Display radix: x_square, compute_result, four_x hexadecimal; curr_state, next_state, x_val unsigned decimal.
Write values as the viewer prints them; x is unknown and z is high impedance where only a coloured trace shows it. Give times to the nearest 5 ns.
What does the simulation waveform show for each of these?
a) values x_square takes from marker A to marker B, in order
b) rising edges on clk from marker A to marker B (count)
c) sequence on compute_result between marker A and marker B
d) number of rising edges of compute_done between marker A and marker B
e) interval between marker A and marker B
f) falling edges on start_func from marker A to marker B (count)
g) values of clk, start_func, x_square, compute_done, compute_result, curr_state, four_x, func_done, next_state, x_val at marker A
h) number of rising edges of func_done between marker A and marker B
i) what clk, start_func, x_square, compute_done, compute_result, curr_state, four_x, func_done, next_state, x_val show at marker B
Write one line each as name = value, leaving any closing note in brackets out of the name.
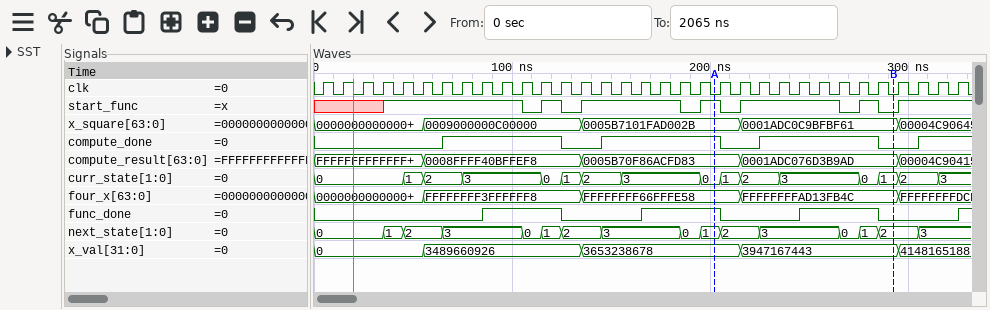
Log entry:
values x_square takes from marker A to marker B, in order = 0005B7101FAD002B, 0001ADC0C9BFBF61
rising edges on clk from marker A to marker B = 9
sequence on compute_result between marker A and marker B = 0005B70F86ACFD83, 0001ADC076D3B9AD
number of rising edges of compute_done between marker A and marker B = 1
interval between marker A and marker B = 90 ns
falling edges on start_func from marker A to marker B = 3
values of clk, start_func, x_square, compute_done, compute_result, curr_state, four_x, func_done, next_state, x_val at marker A = clk=0, start_func=1, x_square=0005B7101FAD002B, compute_done=1, compute_result=0005B70F86ACFD83, curr_state=0, four_x=FFFFFFFF66FFFE58, func_done=1, next_state=1, x_val=3653238678
number of rising edges of func_done between marker A and marker B = 1
what clk, start_func, x_square, compute_done, compute_result, curr_state, four_x, func_done, next_state, x_val show at marker B = clk=0, start_func=0, x_square=0001ADC0C9BFBF61, compute_done=0, compute_result=0001ADC076D3B9AD, curr_state=1, four_x=FFFFFFFFAD13FB4C, func_done=0, next_state=2, x_val=3947167443
